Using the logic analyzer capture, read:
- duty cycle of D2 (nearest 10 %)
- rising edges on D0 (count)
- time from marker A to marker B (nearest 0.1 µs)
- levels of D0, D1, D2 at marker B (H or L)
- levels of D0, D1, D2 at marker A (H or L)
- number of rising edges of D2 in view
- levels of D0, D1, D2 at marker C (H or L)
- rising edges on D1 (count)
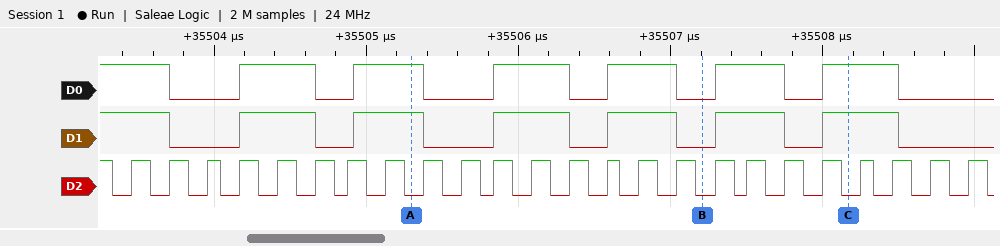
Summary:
50 %
6
1.9 µs
D0=L, D1=L, D2=L
D0=H, D1=H, D2=L
24
D0=H, D1=H, D2=L
6
